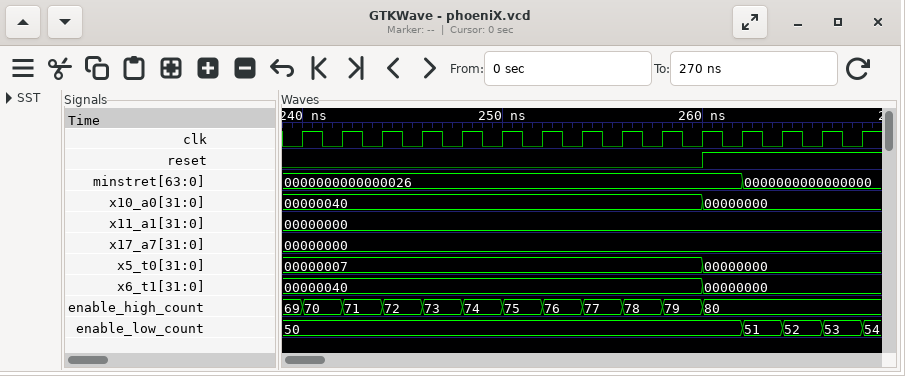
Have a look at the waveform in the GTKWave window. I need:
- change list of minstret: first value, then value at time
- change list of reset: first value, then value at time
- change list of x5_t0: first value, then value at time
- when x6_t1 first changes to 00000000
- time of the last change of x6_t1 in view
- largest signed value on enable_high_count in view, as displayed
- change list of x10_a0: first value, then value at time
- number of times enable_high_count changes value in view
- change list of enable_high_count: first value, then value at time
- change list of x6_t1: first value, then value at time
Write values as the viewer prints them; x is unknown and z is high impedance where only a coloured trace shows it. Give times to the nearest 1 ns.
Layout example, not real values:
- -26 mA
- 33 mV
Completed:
- 0000000000000026, 0000000000000000 at 262 ns
- 0, 1 at 260 ns
- 00000007, 00000000 at 260 ns
- 260 ns
- 260 ns
- 80
- 00000040, 00000000 at 260 ns
- 11
- 69, 70 at 240 ns, 71 at 242 ns, 72 at 244 ns, 73 at 246 ns, 74 at 248 ns, 75 at 250 ns, 76 at 252 ns, 77 at 254 ns, 78 at 256 ns, 79 at 258 ns, 80 at 260 ns
- 00000040, 00000000 at 260 ns
